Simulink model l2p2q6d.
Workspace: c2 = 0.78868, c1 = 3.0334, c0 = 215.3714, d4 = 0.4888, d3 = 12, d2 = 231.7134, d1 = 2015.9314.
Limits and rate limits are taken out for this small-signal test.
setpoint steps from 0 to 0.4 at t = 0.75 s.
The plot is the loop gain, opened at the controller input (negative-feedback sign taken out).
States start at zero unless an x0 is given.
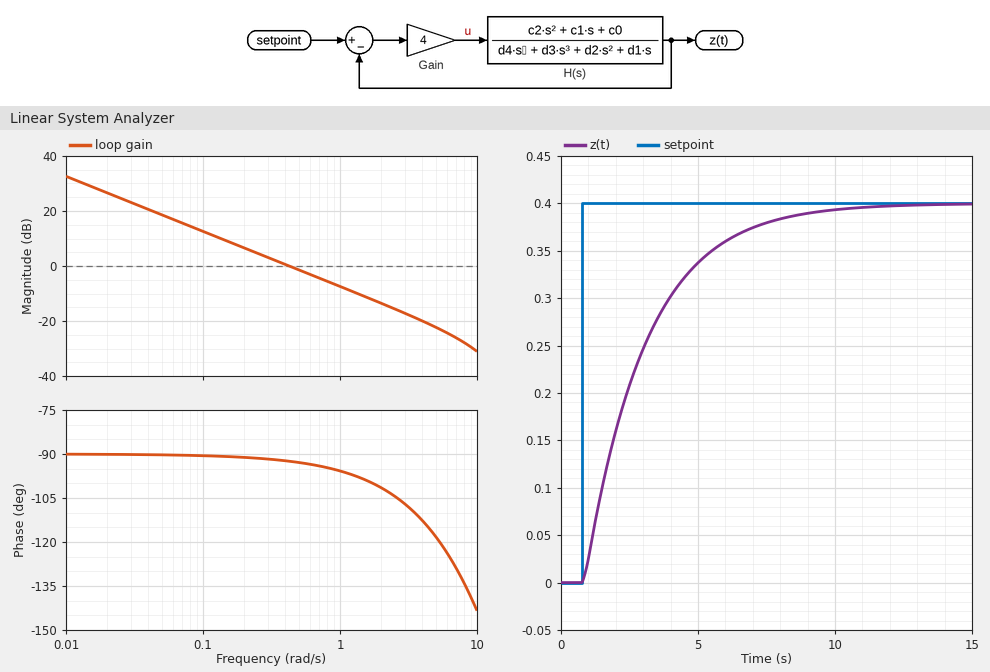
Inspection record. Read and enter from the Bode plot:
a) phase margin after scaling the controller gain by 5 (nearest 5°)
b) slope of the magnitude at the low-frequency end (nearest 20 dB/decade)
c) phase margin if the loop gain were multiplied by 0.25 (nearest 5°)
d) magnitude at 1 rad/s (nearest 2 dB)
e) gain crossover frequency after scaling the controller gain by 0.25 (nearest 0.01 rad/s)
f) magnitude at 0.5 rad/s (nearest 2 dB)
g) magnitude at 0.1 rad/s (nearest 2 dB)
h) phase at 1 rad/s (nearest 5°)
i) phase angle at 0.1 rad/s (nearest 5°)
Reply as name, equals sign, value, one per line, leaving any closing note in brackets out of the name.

phase margin after scaling the controller gain by 5 = 80°
slope of the magnitude at the low-frequency end = -20 dB/decade
phase margin if the loop gain were multiplied by 0.25 = 90°
magnitude at 1 rad/s = -8 dB
gain crossover frequency after scaling the controller gain by 0.25 = 0.11 rad/s
magnitude at 0.5 rad/s = -2 dB
magnitude at 0.1 rad/s = 12 dB
phase at 1 rad/s = -95°
phase angle at 0.1 rad/s = -90°
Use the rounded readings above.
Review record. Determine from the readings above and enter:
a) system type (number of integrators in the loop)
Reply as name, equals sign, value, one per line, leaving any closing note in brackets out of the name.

system type = 1
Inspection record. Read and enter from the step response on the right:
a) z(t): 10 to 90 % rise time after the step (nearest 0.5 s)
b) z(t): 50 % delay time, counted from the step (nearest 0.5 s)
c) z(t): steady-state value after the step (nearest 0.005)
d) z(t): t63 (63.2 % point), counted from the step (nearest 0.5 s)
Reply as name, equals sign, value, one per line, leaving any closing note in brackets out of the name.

z(t): 10 to 90 % rise time after the step = 5.0 s
z(t): 50 % delay time, counted from the step = 1.5 s
z(t): steady-state value after the step = 0.400
z(t): t63 (63.2 % point), counted from the step = 2.5 s
